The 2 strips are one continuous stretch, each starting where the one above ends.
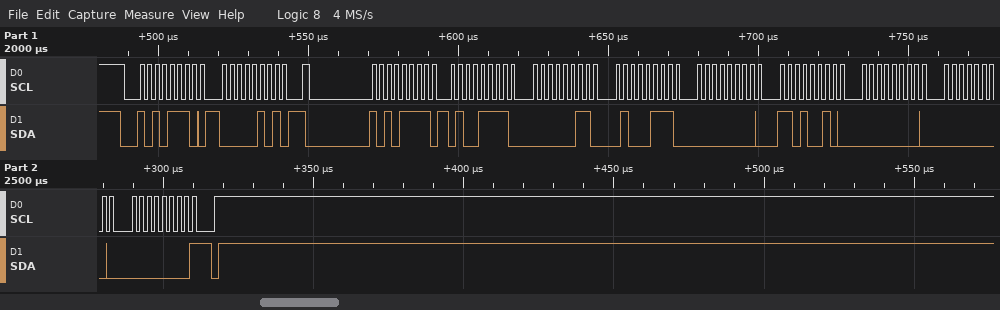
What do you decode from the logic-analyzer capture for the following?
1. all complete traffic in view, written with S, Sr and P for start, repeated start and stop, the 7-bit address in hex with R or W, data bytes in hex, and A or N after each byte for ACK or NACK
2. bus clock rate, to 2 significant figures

S 57W A 05 A Sr 57R A 4F A 03 A 47 A 00 A D2 A 00 A 00 A 00 N P
400 kHz
